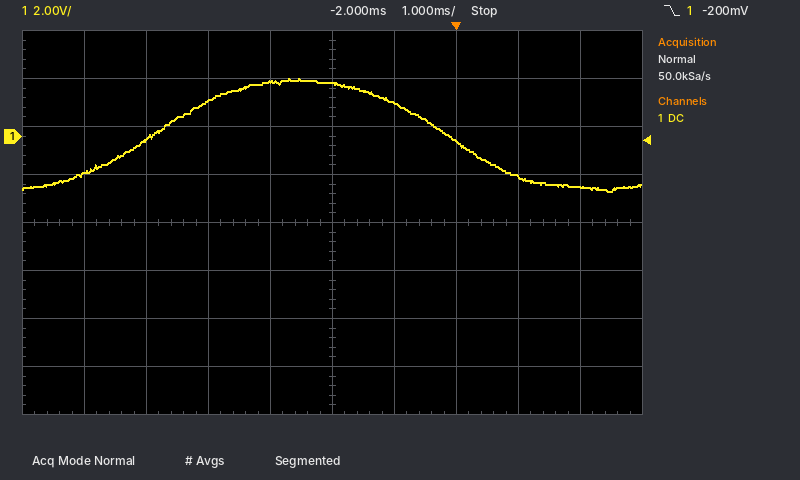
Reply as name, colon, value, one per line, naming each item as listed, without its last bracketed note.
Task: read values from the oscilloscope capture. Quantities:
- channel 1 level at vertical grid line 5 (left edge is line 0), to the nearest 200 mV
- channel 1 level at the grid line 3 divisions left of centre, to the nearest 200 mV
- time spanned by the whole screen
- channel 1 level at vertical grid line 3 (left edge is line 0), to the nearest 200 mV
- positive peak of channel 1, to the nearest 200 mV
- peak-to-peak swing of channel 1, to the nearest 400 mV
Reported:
channel 1 level at vertical grid line 5 (left edge is line 0), to the nearest 200 mV: 2.2 V
channel 1 level at the grid line 3 divisions left of centre, to the nearest 200 mV: -200 mV
time spanned by the whole screen: 10 ms
channel 1 level at vertical grid line 3 (left edge is line 0), to the nearest 200 mV: 1.4 V
positive peak of channel 1, to the nearest 200 mV: 2.4 V
peak-to-peak swing of channel 1, to the nearest 400 mV: 4.8 V
